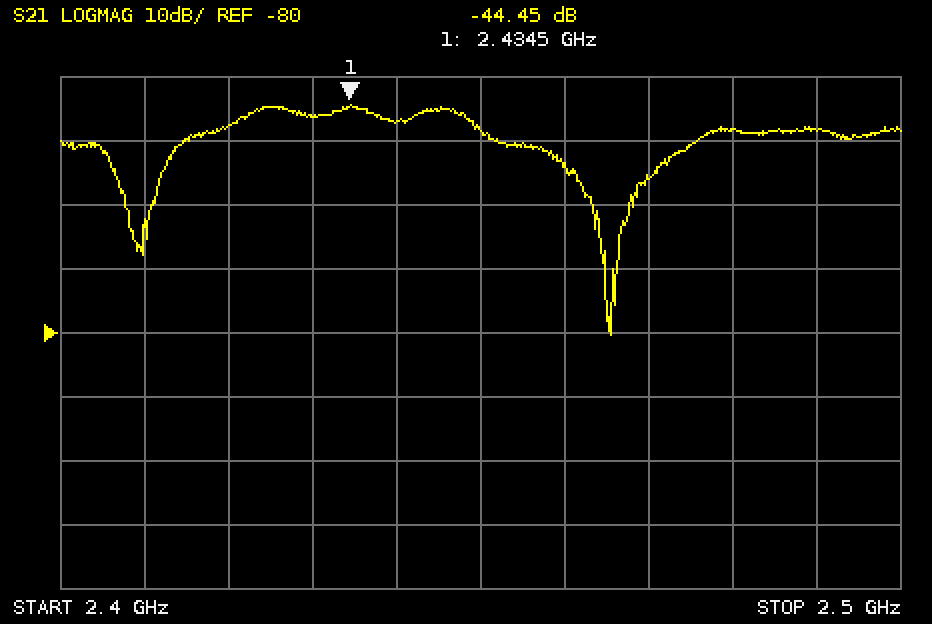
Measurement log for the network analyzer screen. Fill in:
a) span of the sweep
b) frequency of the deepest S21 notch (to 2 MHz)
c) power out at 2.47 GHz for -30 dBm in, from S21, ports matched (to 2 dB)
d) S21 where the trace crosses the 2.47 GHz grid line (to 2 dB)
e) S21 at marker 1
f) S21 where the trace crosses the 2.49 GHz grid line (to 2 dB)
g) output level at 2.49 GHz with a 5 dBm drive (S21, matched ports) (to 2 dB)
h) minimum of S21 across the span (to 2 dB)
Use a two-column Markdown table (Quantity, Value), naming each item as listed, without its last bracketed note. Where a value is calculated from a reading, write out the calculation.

| Quantity | Value |
|---|---|
| span of the sweep | 100 MHz |
| frequency of the deepest S21 notch | 2.466 GHz |
| power out at 2.47 GHz for -30 dBm in, from S21, ports matched | -30 dBm + (-56 dB) = -86 dBm |
| S21 where the trace crosses the 2.47 GHz grid line | -56 dB |
| S21 at marker 1 | -44.45 dB |
| S21 where the trace crosses the 2.49 GHz grid line | -48 dB |
| output level at 2.49 GHz with a 5 dBm drive (S21, matched ports) | 5 dBm + (-48 dB) = -44 dBm |
| minimum of S21 across the span | -80 dB |
